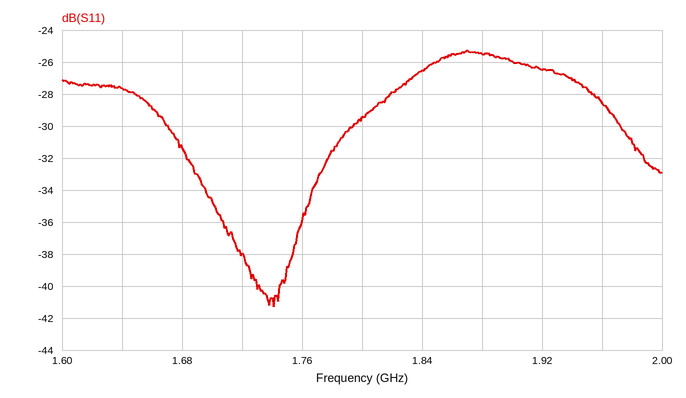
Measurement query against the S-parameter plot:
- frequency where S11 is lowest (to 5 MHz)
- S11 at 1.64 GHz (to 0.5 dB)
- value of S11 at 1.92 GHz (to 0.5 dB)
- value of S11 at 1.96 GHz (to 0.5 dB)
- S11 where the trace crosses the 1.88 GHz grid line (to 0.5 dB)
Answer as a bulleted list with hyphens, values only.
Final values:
- 1.740 GHz
- -27.5 dB
- -26.5 dB
- -28.5 dB
- -25.5 dB
